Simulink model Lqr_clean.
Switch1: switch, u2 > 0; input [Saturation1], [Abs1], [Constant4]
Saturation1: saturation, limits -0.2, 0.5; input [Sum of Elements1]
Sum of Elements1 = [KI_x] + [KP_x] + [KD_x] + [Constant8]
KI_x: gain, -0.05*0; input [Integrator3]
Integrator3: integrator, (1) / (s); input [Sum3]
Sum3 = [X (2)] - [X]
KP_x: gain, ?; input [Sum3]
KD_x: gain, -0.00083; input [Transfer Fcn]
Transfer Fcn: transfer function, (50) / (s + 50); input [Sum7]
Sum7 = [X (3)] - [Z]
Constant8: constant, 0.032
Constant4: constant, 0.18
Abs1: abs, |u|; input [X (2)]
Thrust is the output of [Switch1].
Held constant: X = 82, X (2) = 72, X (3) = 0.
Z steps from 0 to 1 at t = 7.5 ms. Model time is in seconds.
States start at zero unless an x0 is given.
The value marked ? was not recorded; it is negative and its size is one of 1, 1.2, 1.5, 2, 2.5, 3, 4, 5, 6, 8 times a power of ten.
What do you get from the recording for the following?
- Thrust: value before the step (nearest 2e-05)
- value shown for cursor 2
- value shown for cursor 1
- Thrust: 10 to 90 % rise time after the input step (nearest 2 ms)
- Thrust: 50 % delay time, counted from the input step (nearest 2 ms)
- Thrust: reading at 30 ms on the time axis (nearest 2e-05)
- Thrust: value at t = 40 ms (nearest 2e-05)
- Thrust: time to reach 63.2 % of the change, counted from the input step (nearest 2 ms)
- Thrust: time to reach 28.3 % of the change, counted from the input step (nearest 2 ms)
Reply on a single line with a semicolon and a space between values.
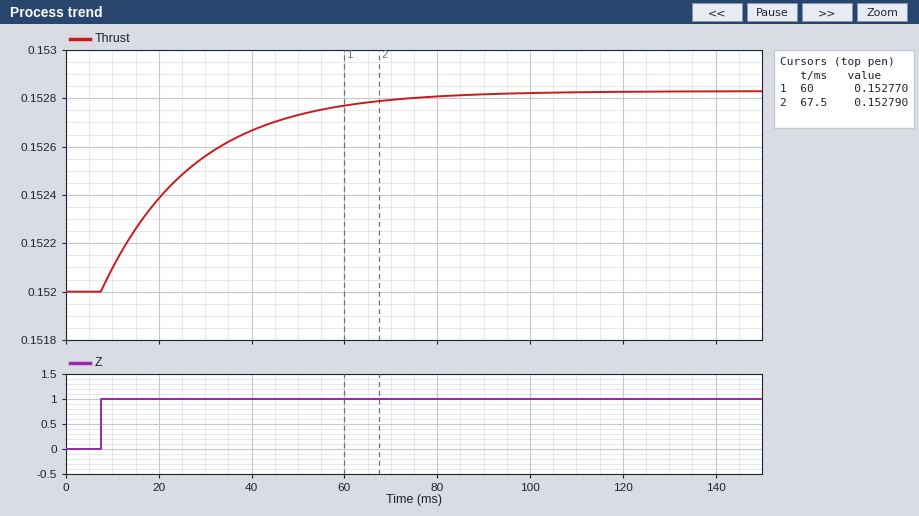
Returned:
0.15200; 0.152790; 0.152770; 44 ms; 14 ms; 0.15256; 0.15266; 20 ms; 6 ms
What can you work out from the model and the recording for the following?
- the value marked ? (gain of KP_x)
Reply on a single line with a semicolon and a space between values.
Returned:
-0.012
